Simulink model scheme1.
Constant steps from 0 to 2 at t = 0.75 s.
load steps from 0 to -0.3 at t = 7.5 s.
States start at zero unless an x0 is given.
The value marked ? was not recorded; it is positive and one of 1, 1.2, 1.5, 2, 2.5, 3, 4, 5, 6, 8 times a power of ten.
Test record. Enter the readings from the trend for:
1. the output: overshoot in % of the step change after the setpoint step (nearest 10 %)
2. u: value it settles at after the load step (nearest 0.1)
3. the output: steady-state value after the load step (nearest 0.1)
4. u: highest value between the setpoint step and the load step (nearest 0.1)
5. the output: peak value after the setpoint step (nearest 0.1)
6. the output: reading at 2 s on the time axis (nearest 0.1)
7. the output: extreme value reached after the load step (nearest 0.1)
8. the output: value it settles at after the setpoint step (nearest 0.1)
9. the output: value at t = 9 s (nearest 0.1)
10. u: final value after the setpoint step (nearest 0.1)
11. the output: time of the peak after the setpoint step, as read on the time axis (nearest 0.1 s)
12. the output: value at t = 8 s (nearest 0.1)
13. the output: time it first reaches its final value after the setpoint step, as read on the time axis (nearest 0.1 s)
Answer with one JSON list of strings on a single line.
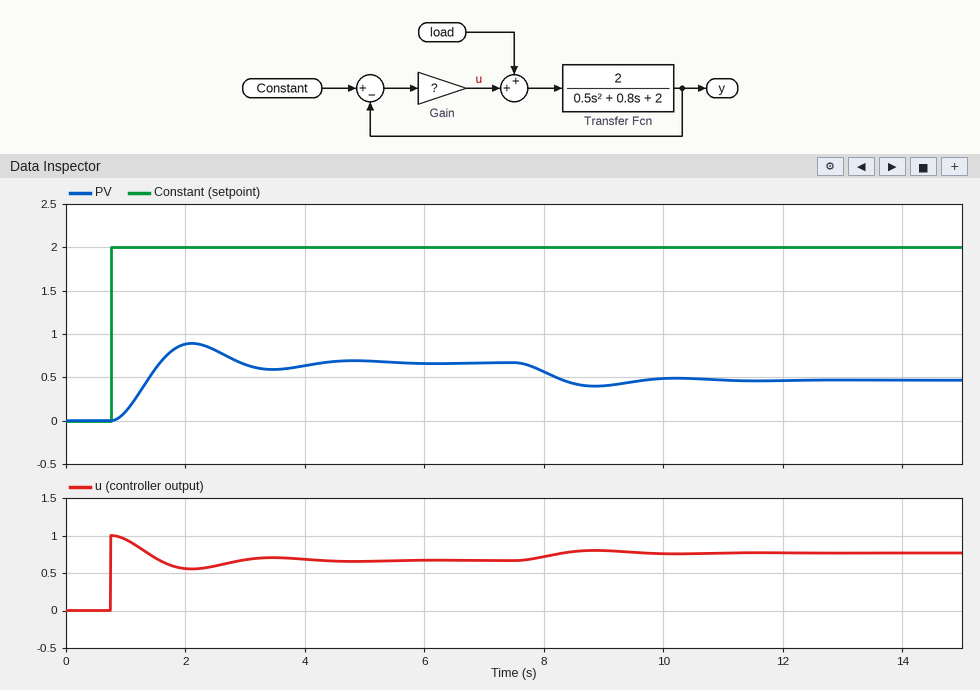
["30 %", "0.8", "0.5", "1.0", "0.9", "0.9", "0.4", "0.7", "0.4", "0.7", "2.1 s", "0.6", "1.6 s"]
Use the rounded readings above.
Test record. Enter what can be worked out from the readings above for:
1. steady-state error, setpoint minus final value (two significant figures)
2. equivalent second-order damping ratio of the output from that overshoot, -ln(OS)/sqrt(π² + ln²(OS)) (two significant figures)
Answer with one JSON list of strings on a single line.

["1.3", "0.36"]
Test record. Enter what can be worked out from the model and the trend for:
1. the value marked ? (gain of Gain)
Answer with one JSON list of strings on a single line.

["0.5"]
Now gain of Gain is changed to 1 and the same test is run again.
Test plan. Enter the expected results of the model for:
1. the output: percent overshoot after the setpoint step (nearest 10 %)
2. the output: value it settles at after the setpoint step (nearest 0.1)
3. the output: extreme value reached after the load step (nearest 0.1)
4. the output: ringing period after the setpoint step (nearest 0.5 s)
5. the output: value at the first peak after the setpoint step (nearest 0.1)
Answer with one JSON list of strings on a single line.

["40 %", "1.0", "0.8", "2.5 s", "1.4"]
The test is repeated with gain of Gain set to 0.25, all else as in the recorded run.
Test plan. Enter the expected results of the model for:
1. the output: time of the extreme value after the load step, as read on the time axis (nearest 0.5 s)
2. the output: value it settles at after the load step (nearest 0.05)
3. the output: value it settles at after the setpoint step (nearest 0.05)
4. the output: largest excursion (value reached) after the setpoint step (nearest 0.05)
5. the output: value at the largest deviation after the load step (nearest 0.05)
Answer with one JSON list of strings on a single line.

["9.0 s", "0.15", "0.40", "0.50", "0.10"]
